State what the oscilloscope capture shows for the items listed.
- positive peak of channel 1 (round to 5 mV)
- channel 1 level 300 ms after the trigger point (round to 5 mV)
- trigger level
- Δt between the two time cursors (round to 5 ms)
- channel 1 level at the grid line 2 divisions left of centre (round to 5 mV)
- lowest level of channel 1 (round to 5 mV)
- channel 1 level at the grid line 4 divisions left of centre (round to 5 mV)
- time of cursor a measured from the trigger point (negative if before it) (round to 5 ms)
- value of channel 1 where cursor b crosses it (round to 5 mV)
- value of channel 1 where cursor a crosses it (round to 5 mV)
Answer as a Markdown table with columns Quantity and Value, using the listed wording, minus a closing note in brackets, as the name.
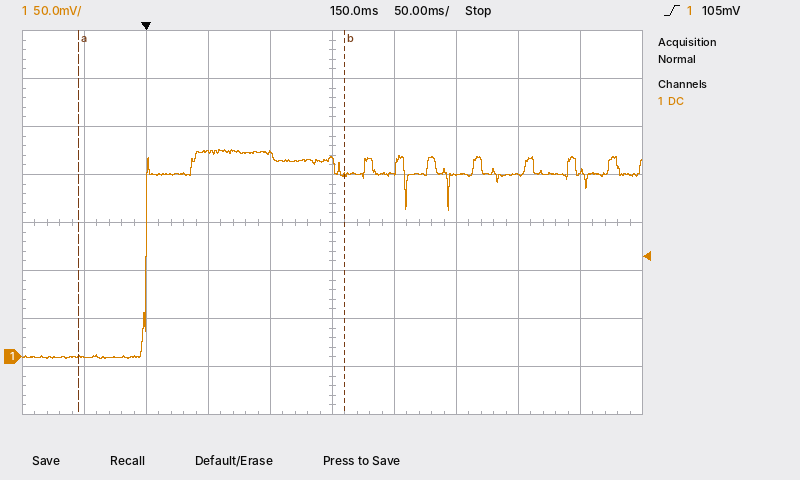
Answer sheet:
| Quantity | Value |
|---|---|
| positive peak of channel 1 | 215 mV |
| channel 1 level 300 ms after the trigger point | 190 mV |
| trigger level | 105 mV |
| Δt between the two time cursors | 215 ms |
| channel 1 level at the grid line 2 divisions left of centre | 215 mV |
| lowest level of channel 1 | 0 mV |
| channel 1 level at the grid line 4 divisions left of centre | 0 mV |
| time of cursor a measured from the trigger point (negative if before it) | -55 ms |
| value of channel 1 where cursor b crosses it | 190 mV |
| value of channel 1 where cursor a crosses it | 0 mV |
